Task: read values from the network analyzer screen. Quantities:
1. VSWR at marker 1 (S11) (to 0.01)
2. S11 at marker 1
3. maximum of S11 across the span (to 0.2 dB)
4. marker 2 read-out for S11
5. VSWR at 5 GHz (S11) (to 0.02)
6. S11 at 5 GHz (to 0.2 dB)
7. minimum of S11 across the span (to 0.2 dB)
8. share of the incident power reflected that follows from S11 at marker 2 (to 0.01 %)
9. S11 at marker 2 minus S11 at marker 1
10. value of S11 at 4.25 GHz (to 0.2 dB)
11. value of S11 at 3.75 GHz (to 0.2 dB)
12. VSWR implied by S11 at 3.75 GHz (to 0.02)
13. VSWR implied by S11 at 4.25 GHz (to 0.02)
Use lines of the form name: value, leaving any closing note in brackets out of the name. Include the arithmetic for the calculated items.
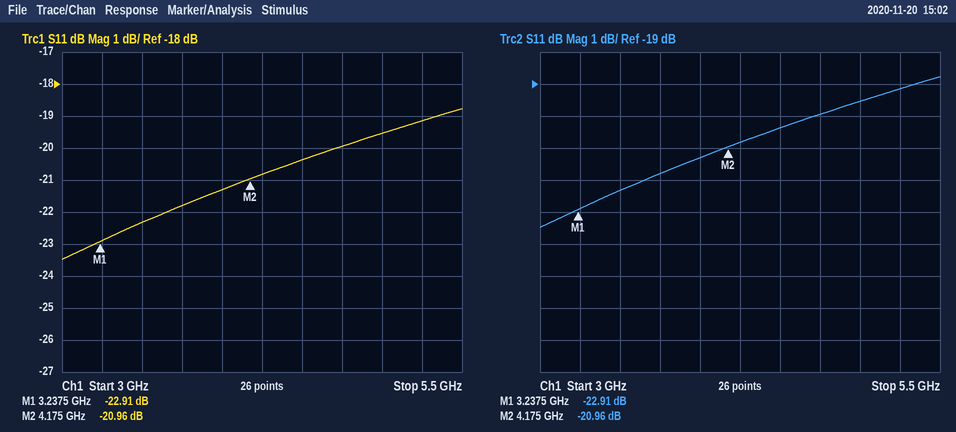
VSWR at marker 1 (S11): (1 + 0.0715)/(1 − 0.0715) ≈ 1.15
S11 at marker 1: -22.91 dB
maximum of S11 across the span: -18.8 dB
marker 2 read-out for S11: -20.96 dB
VSWR at 5 GHz (S11): |Γ| = 10^(-19.6/20) = 0.1047; VSWR = (1 + 0.1047)/(1 − 0.1047) ≈ 1.23, so 1.24 to the nearest 0.02
S11 at 5 GHz: -19.6 dB
minimum of S11 across the span: -23.4 dB
share of the incident power reflected that follows from S11 at marker 2: 10^(-20.96/10) ≈ 0.80 %
S11 at marker 2 minus S11 at marker 1: -20.96 − (-22.91) = 1.95 dB
value of S11 at 4.25 GHz: -20.8 dB
value of S11 at 3.75 GHz: -21.8 dB
VSWR implied by S11 at 3.75 GHz: |Γ| = 10^(-21.8/20) = 0.0813; VSWR = (1 + 0.0813)/(1 − 0.0813) ≈ 1.18
VSWR implied by S11 at 4.25 GHz: |Γ| = 10^(-20.8/20) = 0.0912; VSWR = (1 + 0.0912)/(1 − 0.0912) ≈ 1.20
